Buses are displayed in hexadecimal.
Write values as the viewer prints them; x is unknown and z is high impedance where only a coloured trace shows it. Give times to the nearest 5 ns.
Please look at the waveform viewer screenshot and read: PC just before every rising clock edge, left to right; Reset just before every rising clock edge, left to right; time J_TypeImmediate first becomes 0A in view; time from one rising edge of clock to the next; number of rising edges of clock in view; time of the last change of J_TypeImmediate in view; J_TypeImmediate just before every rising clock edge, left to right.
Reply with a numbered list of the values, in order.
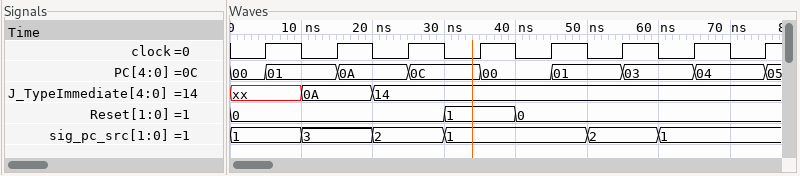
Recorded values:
1. 00, 01, 0A, 0C, 00, 01, 03, 04
2. 0, 0, 0, 1, 0, 0, 0, 0
3. 10 ns
4. 10 ns
5. 8
6. 20 ns
7. xx, 0A, 14, 14, 14, 14, 14, 14
